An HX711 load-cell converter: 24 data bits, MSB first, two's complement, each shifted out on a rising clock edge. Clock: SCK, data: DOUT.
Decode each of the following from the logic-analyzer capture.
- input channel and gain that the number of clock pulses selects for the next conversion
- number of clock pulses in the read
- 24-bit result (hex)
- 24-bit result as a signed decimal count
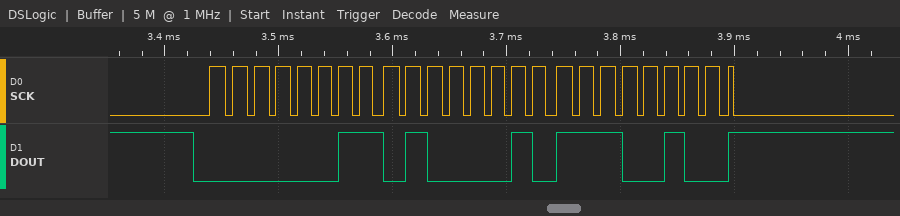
channel A, gain 128
25
0x0342E4
213732
